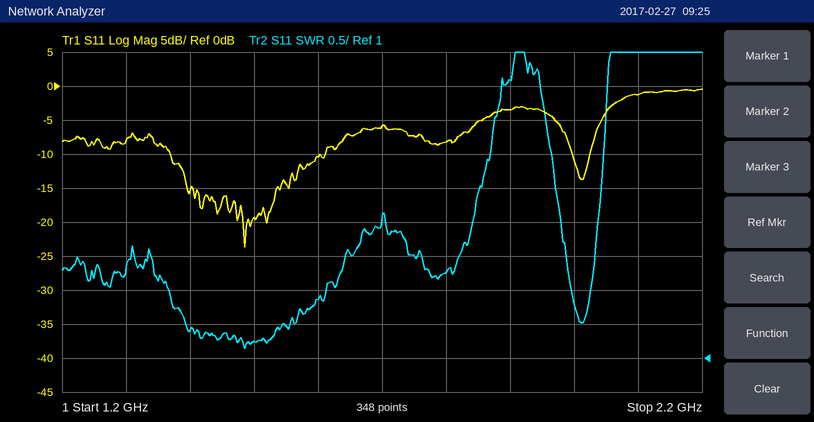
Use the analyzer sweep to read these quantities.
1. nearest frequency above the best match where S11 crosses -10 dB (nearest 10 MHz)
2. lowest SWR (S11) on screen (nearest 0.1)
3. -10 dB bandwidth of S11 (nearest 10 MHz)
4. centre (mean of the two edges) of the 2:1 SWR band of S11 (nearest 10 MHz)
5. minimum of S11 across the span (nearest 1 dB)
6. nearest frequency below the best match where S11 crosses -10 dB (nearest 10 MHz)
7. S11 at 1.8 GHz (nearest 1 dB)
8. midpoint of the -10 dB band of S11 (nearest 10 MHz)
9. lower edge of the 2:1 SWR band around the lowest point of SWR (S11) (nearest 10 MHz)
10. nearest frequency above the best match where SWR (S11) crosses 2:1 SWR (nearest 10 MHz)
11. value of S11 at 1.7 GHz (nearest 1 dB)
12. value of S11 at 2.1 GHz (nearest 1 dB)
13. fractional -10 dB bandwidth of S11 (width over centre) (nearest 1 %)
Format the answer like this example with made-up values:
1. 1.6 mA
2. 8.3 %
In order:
1. 1.61 GHz
2. 1.1
3. 240 MHz
4. 1.49 GHz
5. -24 dB
6. 1.37 GHz
7. -8 dB
8. 1.49 GHz
9. 1.37 GHz
10. 1.61 GHz
11. -6 dB
12. -1 dB
13. 16 %
